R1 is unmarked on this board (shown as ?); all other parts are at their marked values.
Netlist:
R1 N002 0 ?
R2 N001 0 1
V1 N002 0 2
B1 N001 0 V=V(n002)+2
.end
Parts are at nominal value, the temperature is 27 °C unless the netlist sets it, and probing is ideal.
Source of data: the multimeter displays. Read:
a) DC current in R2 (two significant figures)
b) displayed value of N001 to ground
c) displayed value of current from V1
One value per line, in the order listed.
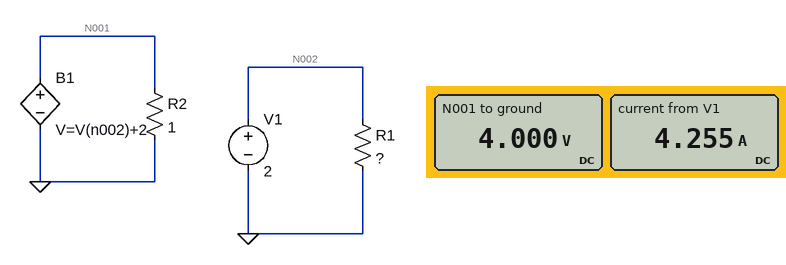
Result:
4.0 A
4.000 V
4.255 A
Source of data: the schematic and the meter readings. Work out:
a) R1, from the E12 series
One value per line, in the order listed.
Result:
0.47 Ω
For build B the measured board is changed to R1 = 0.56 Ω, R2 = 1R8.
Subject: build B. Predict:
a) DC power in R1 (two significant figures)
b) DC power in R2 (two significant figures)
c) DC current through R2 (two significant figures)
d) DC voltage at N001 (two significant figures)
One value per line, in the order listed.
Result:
7.1 W
8.9 W
2.2 A
4.0 V
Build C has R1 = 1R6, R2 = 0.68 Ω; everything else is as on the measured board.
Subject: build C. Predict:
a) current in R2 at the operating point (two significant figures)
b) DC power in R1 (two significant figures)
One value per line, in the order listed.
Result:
5.9 A
2.5 W
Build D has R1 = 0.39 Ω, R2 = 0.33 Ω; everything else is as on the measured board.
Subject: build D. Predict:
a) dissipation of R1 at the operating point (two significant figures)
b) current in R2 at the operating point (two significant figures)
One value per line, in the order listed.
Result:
10 W
12 A
